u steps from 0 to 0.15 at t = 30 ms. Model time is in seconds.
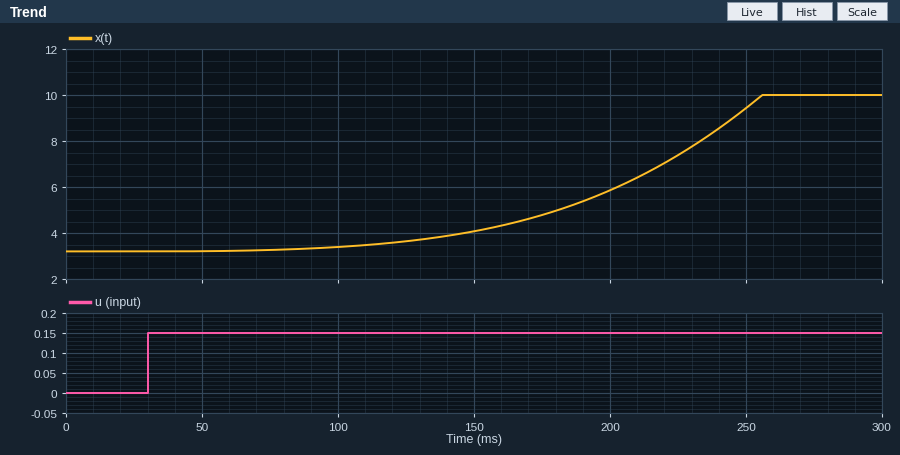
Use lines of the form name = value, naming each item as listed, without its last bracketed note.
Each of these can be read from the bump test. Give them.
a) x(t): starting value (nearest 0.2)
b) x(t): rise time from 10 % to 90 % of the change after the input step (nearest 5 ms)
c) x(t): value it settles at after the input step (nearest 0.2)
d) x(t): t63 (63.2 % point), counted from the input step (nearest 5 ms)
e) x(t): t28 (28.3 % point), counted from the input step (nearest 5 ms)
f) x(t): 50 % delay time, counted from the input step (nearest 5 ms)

x(t): starting value = 3.2
x(t): rise time from 10 % to 90 % of the change after the input step = 110 ms
x(t): value it settles at after the input step = 10.0
x(t): t63 (63.2 % point), counted from the input step = 195 ms
x(t): t28 (28.3 % point), counted from the input step = 155 ms
x(t): 50 % delay time, counted from the input step = 185 ms
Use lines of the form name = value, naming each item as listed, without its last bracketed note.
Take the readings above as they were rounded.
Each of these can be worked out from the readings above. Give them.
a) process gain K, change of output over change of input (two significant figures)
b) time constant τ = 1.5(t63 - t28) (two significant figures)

process gain K, change of output over change of input = 45
time constant τ = 1.5(t63 - t28) = 60 ms
